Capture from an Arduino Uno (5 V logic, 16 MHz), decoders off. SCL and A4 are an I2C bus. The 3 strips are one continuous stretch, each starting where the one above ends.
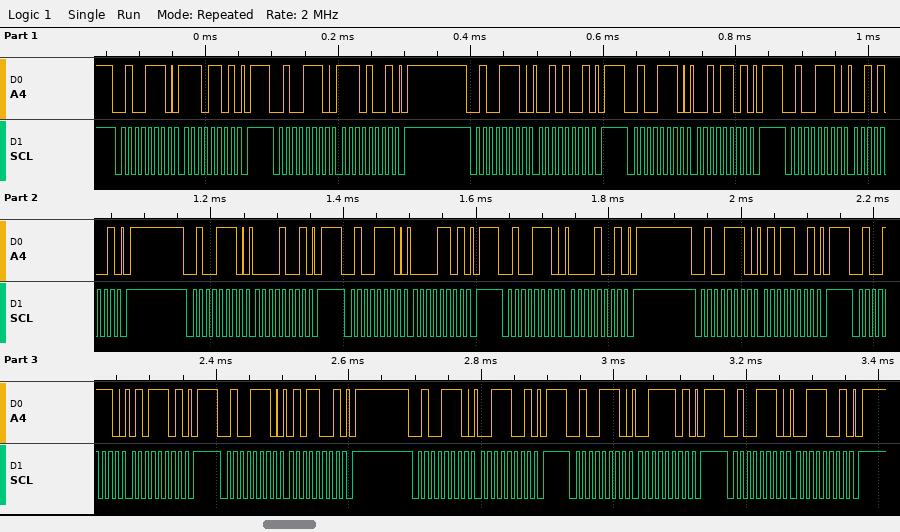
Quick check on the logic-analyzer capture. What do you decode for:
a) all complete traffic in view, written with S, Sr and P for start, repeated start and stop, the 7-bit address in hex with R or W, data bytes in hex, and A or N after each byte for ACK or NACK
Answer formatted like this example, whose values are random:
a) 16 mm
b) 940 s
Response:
a) S 27W A ED A P S 27W A E9 A P S 27W A 29 A P S 27W A 2D A P S 27W A 29 A P S 27W A 09 A P S 27W A 0D A P S 27W A 09 A P S 27W A 59 A P S 27W A 5D A P S 27W A 59 A P S 27W A 39 A P S 27W A 3D A P S 27W A 39 A P
